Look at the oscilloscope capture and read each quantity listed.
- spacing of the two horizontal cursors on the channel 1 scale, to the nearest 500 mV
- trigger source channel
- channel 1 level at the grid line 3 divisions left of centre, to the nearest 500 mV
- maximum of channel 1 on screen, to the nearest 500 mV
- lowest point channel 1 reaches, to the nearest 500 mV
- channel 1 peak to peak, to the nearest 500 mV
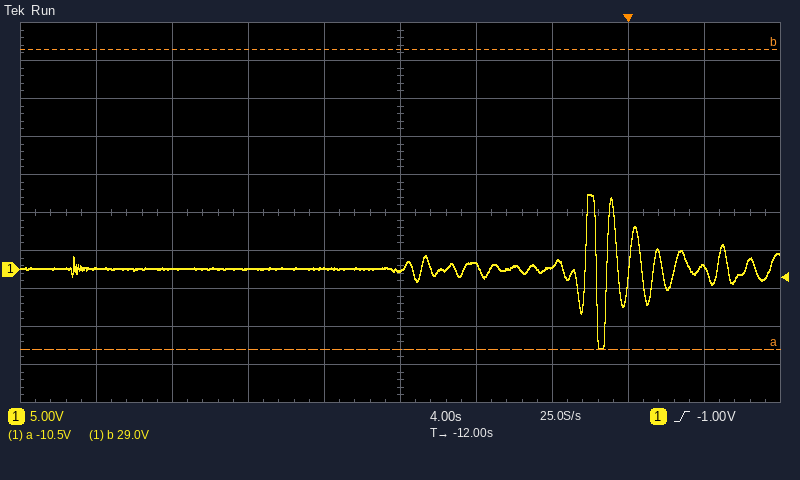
39.5 V
channel 1
0.0 V
10.0 V
-10.5 V
20.5 V
